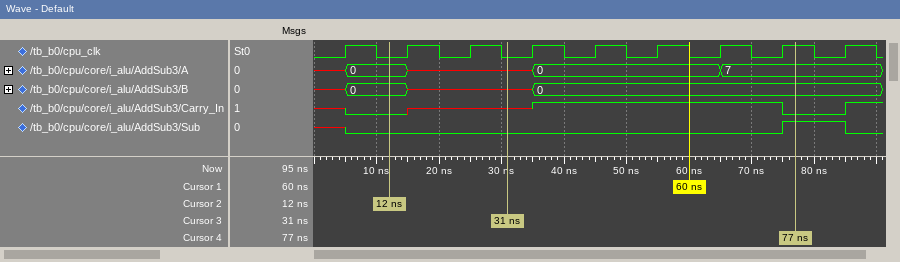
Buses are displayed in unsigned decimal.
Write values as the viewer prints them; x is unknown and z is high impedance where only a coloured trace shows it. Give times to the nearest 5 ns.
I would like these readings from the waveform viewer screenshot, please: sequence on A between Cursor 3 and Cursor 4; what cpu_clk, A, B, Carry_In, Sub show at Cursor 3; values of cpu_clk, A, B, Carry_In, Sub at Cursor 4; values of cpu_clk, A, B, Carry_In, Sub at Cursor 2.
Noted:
x, 0, 7
cpu_clk=0, A=x, B=x, Carry_In=x, Sub=0
cpu_clk=1, A=7, B=0, Carry_In=0, Sub=1
cpu_clk=0, A=0, B=0, Carry_In=0, Sub=0
